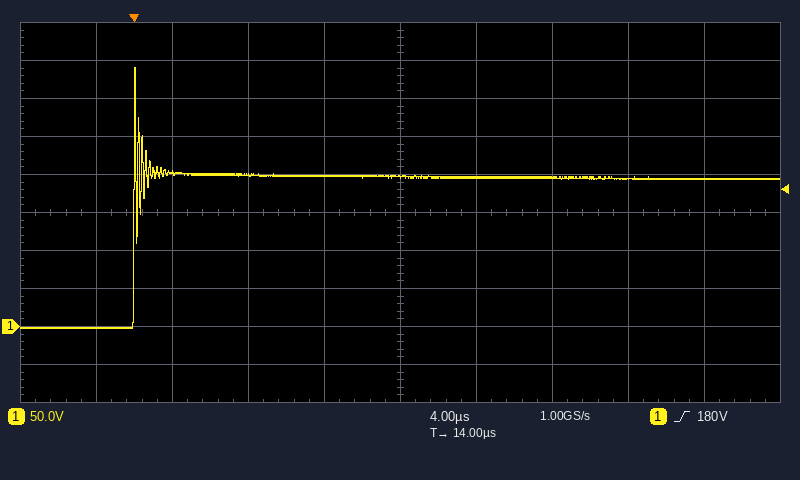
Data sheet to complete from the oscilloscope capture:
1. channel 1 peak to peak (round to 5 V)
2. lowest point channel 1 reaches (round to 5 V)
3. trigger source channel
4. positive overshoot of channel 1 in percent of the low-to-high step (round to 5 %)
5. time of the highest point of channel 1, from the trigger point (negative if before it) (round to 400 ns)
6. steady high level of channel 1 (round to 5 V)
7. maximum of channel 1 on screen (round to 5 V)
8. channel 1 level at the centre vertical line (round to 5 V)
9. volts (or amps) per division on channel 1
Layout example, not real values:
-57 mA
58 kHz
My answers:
345 V
-5 V
channel 1
75 %
0.0 µs
195 V
340 V
195 V
50 V
